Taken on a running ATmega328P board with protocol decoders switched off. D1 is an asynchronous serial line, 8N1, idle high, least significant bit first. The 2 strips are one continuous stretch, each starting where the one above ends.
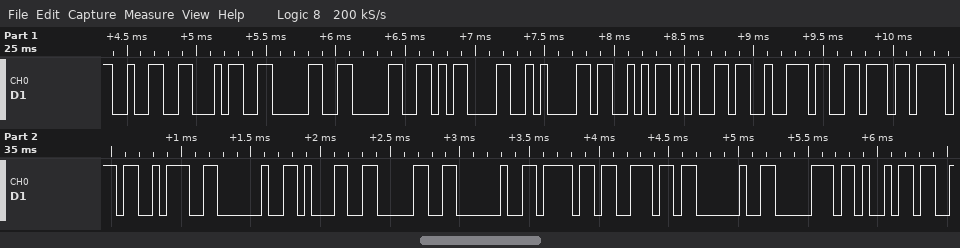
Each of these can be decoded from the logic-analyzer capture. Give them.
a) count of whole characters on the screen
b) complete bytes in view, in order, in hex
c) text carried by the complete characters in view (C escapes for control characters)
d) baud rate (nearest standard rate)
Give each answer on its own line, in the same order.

21
32 34 30 30 0D 0A 53 65 72 76 6F 3A 20 31 30 20 6F 6E 20 70 69
"2400\r\nServo: 10 on pi"
19200 baud
